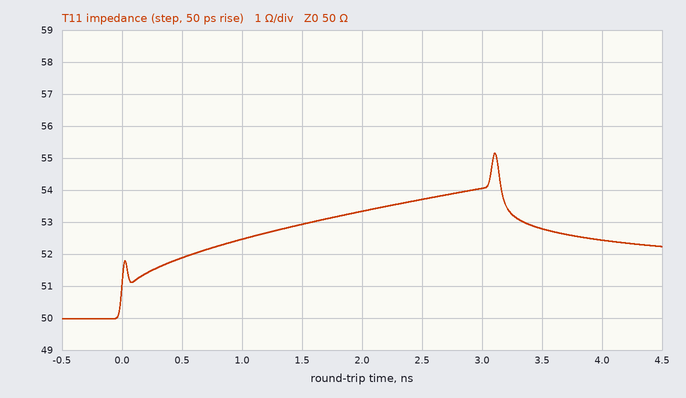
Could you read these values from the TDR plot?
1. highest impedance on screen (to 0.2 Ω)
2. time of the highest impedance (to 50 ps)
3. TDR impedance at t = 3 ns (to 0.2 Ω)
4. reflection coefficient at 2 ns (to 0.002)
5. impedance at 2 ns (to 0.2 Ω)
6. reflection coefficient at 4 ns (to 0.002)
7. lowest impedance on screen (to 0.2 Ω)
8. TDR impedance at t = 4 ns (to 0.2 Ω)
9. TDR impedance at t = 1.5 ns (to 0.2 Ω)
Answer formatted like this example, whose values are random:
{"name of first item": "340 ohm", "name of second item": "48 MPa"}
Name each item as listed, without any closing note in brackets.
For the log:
{"highest impedance on screen": "55.2 Ω", "time of the highest impedance": "3.10 ns", "TDR impedance at t = 3 ns": "54.0 Ω", "reflection coefficient at 2 ns": "+0.032", "impedance at 2 ns": "53.4 Ω", "reflection coefficient at 4 ns": "+0.024", "lowest impedance on screen": "50.0 Ω", "TDR impedance at t = 4 ns": "52.4 Ω", "TDR impedance at t = 1.5 ns": "53.0 Ω"}
